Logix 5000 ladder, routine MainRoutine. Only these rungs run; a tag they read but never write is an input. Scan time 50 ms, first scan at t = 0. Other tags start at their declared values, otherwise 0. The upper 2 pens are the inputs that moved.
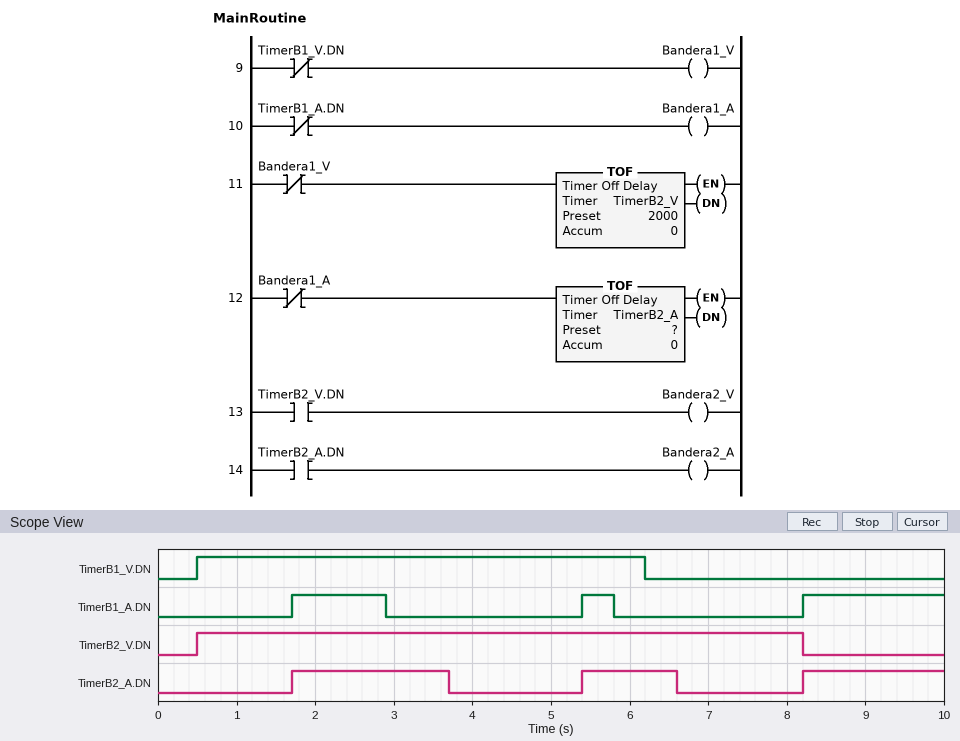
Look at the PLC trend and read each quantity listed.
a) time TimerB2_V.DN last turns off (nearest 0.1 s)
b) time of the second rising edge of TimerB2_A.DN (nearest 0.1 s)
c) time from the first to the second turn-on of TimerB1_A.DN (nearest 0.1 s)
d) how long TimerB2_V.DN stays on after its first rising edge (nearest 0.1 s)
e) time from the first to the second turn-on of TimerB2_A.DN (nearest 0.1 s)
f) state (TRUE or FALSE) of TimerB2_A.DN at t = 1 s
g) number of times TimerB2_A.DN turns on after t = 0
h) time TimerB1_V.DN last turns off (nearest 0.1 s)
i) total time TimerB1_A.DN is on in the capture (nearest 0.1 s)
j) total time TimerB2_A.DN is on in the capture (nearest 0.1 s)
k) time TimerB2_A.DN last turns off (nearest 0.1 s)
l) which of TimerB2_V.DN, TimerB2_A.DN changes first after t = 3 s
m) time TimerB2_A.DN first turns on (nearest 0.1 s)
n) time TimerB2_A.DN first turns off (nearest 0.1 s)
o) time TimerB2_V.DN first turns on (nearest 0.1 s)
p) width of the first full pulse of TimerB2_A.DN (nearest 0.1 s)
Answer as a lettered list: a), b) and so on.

a) 8.2 s
b) 5.4 s
c) 3.7 s
d) 7.7 s
e) 3.7 s
f) FALSE
g) 3
h) 6.2 s
i) 3.4 s
j) 5.0 s
k) 6.6 s
l) TimerB2_A.DN
m) 1.7 s
n) 3.7 s
o) 0.5 s
p) 2.0 s
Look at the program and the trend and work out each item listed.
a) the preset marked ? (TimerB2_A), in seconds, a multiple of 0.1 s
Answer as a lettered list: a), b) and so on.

a) 0.8 s
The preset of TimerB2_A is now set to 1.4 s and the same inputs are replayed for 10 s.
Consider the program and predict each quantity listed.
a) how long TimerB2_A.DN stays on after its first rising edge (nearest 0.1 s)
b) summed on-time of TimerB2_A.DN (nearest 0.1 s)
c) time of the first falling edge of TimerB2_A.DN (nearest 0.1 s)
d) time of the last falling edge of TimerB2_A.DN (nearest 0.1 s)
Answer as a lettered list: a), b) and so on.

a) 2.6 s
b) 6.2 s
c) 4.3 s
d) 7.2 s
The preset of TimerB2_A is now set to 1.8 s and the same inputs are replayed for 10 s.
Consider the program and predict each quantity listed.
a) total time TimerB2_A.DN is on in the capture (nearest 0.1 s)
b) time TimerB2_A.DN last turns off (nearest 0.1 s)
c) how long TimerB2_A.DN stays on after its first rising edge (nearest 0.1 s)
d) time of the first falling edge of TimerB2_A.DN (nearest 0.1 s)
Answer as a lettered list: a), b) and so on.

a) 7.0 s
b) 7.6 s
c) 3.0 s
d) 4.7 s
